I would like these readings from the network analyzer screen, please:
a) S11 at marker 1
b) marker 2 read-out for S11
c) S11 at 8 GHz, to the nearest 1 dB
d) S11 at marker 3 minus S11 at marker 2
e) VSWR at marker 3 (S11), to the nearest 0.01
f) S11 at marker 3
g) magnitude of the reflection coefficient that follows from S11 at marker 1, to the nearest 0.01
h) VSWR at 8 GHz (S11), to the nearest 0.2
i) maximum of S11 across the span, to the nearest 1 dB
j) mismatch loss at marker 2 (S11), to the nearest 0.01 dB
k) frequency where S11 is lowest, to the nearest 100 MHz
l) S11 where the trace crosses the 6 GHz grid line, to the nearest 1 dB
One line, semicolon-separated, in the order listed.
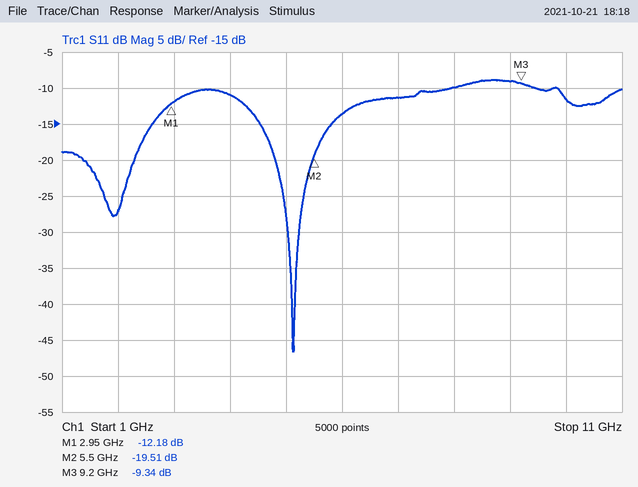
-12.18 dB; -19.51 dB; -10 dB; 10.17 dB; 2.04; -9.34 dB; 0.25; 2.0; -9 dB; 0.05 dB; 5.1 GHz; -14 dB
